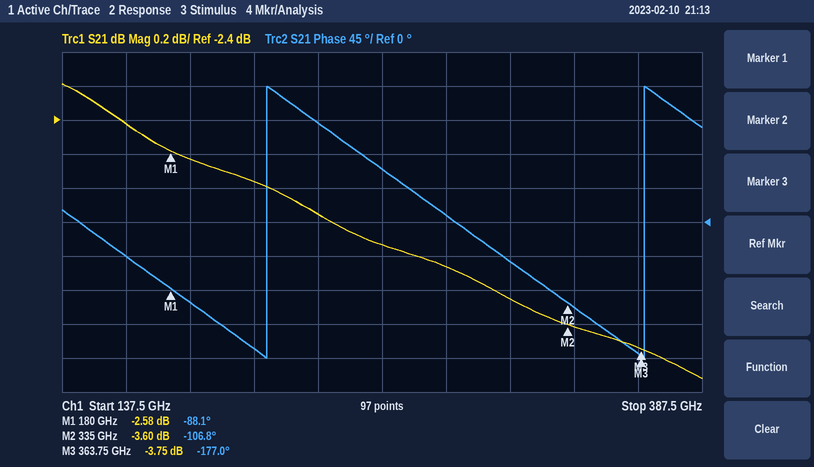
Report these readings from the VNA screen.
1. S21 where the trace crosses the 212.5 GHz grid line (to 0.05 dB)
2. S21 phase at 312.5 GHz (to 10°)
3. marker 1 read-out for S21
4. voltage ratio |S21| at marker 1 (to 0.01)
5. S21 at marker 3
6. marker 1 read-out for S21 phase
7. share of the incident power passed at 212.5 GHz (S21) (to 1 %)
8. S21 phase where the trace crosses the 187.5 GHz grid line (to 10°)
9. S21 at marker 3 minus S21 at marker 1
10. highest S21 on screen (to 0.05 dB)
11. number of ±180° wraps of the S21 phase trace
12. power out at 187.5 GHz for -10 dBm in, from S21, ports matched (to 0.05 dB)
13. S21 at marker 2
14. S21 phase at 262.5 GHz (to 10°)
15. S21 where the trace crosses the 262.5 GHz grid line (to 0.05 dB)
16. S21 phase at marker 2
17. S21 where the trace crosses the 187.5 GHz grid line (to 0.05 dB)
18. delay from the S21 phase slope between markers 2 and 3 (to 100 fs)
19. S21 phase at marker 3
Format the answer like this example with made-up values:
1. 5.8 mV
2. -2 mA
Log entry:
1. -2.75 dB
2. -50°
3. -2.58 dB
4. 0.74
5. -3.75 dB
6. -88.1°
7. 53 %
8. -110°
9. -1.17 dB
10. -2.20 dB
11. 2
12. -12.65 dBm
13. -3.60 dB
14. 70°
15. -3.15 dB
16. -106.8°
17. -2.65 dB
18. 6.8 ps
19. -177.0°
